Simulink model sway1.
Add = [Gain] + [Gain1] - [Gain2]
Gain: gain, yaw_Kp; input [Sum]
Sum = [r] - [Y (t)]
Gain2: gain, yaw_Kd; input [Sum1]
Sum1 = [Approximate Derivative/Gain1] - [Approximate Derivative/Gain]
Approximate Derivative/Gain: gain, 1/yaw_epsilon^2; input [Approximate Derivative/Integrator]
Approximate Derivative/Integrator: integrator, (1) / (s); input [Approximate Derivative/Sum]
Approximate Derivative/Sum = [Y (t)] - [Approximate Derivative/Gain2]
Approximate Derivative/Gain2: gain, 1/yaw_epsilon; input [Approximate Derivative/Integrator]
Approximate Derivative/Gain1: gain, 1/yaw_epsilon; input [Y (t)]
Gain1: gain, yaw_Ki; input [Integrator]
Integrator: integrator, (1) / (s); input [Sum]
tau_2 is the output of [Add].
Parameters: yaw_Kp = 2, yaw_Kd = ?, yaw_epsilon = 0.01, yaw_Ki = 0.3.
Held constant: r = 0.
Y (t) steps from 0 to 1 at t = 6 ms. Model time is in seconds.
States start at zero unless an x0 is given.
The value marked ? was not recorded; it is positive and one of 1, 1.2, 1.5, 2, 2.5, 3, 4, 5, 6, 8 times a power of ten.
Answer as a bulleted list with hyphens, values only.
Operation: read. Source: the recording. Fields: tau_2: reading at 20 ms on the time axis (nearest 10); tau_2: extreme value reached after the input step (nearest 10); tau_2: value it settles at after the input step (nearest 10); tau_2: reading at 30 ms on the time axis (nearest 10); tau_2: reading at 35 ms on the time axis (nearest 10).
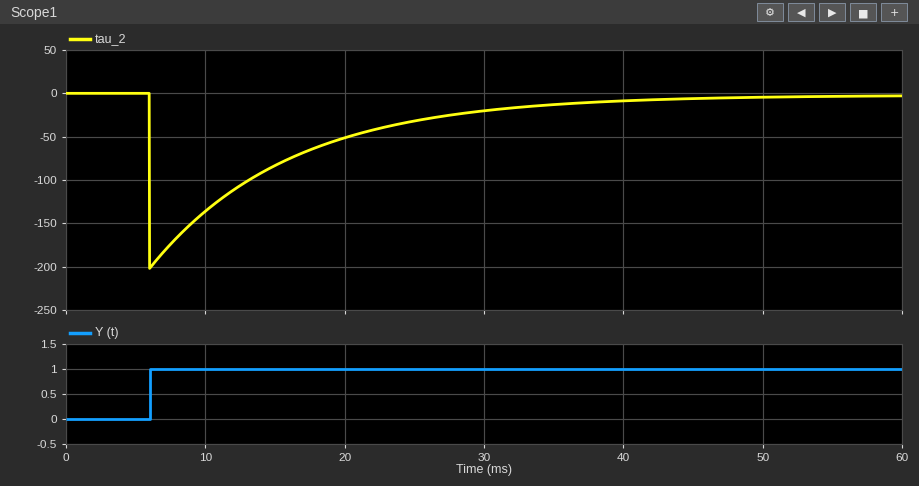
- -50
- -200
- 0
- -20
- -10
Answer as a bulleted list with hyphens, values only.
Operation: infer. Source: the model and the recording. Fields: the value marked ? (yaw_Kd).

- 2
